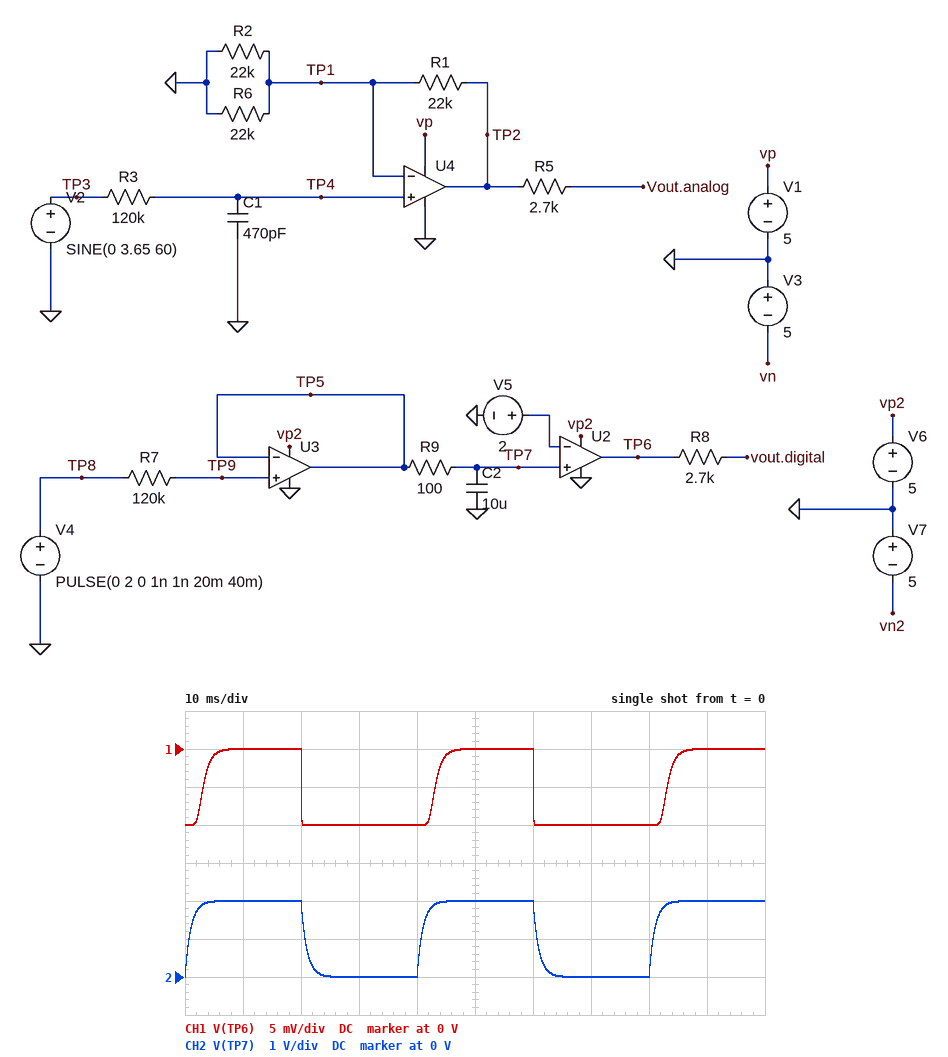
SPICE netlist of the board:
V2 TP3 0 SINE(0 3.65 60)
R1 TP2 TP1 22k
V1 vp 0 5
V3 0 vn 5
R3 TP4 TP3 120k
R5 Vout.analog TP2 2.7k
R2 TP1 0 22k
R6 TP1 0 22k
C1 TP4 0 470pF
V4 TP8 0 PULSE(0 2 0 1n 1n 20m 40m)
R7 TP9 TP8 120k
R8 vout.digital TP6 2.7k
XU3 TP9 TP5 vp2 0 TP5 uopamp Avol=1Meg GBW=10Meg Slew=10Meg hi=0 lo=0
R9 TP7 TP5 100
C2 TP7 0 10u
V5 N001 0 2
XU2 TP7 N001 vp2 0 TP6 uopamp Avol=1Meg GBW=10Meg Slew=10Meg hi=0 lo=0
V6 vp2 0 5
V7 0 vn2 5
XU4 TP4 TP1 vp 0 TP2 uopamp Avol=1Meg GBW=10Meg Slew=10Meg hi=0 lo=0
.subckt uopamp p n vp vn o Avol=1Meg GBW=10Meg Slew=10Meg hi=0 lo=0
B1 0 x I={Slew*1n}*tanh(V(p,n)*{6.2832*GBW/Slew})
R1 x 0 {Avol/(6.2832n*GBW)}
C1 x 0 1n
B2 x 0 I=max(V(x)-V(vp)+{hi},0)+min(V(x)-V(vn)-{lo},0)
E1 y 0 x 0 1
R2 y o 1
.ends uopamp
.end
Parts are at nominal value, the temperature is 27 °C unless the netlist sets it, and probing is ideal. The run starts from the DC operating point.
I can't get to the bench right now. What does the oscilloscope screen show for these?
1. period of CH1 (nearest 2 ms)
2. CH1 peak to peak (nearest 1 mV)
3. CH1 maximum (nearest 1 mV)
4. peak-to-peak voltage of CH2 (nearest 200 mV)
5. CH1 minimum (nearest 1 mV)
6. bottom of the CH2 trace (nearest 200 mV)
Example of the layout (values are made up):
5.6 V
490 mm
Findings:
40 ms
10 mV
0 V
2.0 V
-10 mV
0 V
